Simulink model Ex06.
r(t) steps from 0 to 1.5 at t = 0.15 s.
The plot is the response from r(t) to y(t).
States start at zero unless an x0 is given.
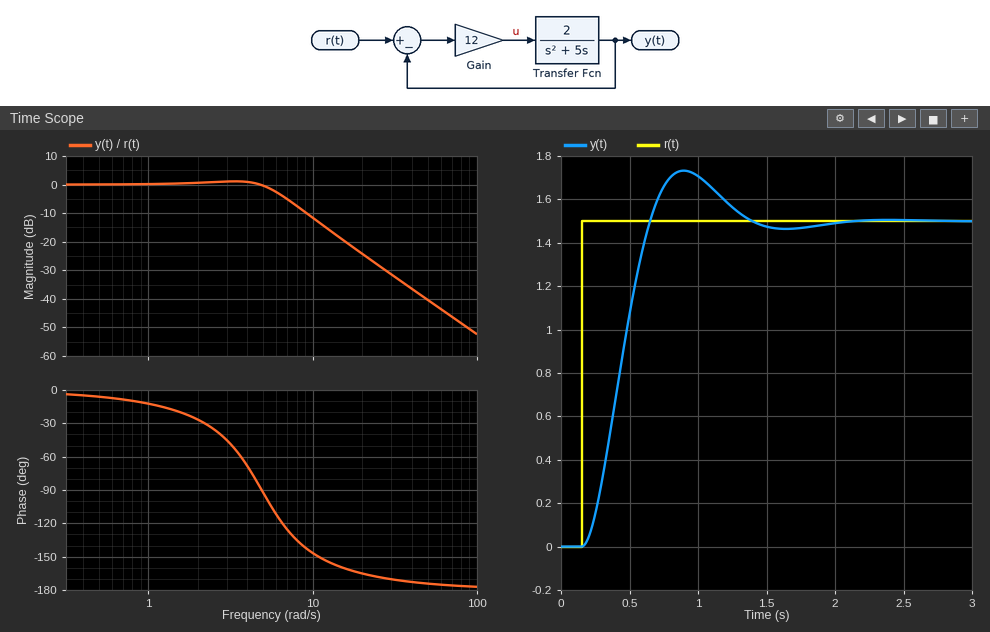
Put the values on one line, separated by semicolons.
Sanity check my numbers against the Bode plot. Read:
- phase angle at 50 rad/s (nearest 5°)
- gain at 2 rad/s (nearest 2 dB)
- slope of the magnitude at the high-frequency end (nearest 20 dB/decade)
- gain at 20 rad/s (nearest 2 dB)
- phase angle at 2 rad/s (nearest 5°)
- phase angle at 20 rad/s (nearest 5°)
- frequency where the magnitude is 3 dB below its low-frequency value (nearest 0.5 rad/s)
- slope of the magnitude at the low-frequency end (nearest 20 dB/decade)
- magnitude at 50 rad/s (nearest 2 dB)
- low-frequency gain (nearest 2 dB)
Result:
-175°; 0 dB; -40 dB/decade; -24 dB; -25°; -165°; 6.0 rad/s; 0 dB/decade; -40 dB; 0 dB
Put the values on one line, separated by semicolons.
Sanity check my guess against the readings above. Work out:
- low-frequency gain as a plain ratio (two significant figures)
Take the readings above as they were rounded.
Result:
1.0
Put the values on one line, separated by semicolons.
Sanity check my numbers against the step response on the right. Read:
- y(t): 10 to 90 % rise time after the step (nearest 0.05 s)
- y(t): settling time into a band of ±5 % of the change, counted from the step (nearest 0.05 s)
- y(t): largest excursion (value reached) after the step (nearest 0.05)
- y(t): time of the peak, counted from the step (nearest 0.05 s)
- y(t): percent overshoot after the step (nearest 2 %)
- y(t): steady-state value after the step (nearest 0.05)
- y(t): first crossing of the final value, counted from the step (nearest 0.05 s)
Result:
0.35 s; 1.10 s; 1.75; 0.75 s; 16 %; 1.50; 0.50 s
